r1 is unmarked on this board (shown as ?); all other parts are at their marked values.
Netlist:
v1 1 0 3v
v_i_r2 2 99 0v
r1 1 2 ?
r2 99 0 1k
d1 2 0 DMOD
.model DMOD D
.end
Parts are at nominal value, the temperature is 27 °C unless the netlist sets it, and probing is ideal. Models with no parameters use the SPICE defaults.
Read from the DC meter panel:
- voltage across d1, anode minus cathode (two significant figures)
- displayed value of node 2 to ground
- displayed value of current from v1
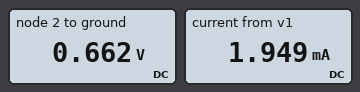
660 mV
0.662 V
1.949 mA
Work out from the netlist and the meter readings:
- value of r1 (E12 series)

1.2 kΩ
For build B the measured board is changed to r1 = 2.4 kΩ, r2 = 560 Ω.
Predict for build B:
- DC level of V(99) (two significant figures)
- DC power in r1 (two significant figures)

560 mV
2.5 mW
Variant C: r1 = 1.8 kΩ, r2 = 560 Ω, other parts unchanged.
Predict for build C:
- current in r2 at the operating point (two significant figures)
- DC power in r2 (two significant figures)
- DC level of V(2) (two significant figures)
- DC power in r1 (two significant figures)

1.1 mA
680 µW
620 mV
3.2 mW
